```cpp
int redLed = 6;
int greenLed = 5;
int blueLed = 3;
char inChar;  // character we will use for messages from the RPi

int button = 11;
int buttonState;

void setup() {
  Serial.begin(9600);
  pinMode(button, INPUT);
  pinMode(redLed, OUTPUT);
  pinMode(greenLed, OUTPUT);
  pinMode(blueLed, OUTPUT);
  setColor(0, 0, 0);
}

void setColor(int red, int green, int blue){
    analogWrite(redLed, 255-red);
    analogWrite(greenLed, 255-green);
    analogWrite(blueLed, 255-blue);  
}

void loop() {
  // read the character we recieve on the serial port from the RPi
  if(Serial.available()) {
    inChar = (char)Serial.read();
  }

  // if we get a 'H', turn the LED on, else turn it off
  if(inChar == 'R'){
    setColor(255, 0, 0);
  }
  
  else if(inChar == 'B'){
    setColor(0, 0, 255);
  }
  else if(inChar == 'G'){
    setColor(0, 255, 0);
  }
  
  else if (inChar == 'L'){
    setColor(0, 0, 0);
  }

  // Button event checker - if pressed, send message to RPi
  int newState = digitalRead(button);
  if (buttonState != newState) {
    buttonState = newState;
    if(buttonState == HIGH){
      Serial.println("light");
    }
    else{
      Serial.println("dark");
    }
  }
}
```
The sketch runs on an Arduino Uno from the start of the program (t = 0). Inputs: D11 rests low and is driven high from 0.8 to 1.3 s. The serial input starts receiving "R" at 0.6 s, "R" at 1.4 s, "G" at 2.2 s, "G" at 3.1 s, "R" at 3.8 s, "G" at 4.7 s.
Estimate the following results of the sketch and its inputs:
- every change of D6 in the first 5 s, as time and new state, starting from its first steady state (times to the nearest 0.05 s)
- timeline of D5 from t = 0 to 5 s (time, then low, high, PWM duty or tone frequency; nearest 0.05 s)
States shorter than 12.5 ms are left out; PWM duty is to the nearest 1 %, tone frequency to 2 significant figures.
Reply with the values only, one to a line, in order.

0 s high; 0.6 s low; 2.2 s high; 3.8 s low; 4.7 s high
0 s high; 2.2 s low; 3.8 s high; 4.7 s low
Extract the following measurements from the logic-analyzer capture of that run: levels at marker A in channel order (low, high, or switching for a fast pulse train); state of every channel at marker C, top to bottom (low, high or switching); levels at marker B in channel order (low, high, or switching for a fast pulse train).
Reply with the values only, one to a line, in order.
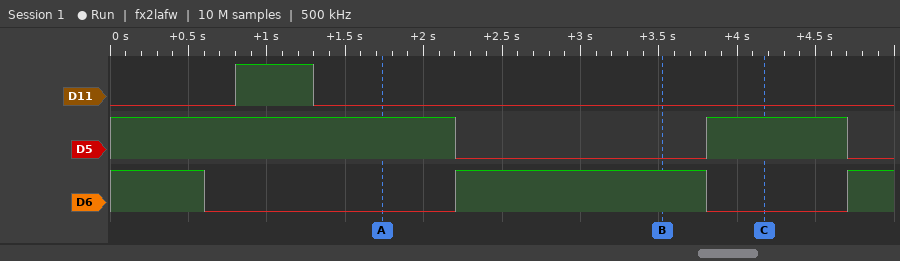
D11 low, D5 high, D6 low
D11 low, D5 high, D6 low
D11 low, D5 low, D6 high
